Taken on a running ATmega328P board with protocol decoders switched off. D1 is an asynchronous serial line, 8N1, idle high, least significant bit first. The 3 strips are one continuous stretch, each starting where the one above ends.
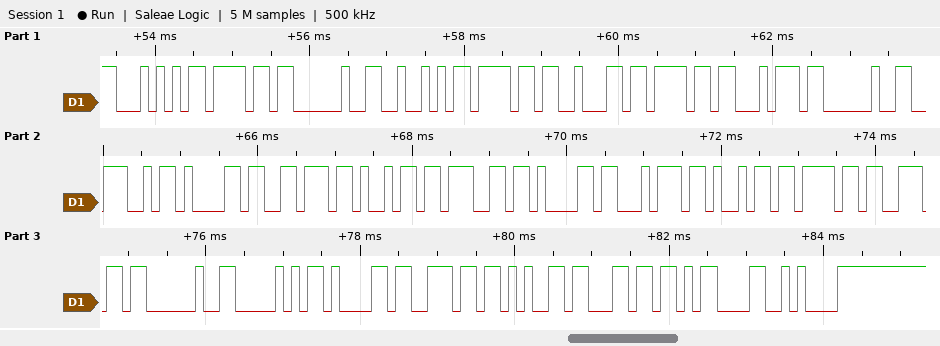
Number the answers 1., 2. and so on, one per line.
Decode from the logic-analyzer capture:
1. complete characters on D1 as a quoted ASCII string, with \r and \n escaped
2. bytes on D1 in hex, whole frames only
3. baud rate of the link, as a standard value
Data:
1. "To Robot Navigation Panel\r\n"
2. 54 6F 20 52 6F 62 6F 74 20 4E 61 76 69 67 61 74 69 6F 6E 20 50 61 6E 65 6C 0D 0A
3. 9600 baud
